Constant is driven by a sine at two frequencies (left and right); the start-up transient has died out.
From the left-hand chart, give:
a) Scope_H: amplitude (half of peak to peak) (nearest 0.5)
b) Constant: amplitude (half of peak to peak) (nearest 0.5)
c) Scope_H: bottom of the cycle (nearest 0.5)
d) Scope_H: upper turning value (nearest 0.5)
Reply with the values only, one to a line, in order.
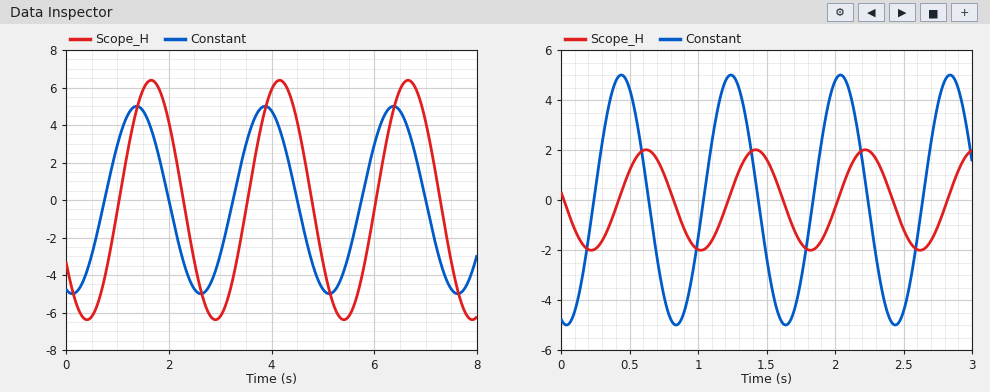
6.5
5.0
-6.5
6.5
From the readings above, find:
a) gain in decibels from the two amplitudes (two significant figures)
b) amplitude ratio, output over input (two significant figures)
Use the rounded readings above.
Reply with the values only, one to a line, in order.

2.3 dB
1.3
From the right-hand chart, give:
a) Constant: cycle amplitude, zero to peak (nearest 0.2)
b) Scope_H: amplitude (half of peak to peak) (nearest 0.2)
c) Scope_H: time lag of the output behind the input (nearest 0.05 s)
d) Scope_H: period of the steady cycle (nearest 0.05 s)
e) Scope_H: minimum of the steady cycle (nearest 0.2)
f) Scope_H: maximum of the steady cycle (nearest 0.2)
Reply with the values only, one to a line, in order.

5.0
2.0
0.20 s
0.80 s
-2.0
2.0
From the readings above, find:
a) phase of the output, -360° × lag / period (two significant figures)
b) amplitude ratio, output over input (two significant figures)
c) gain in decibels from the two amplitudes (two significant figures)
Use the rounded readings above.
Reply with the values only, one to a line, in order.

-90°
0.40
-8.0 dB
